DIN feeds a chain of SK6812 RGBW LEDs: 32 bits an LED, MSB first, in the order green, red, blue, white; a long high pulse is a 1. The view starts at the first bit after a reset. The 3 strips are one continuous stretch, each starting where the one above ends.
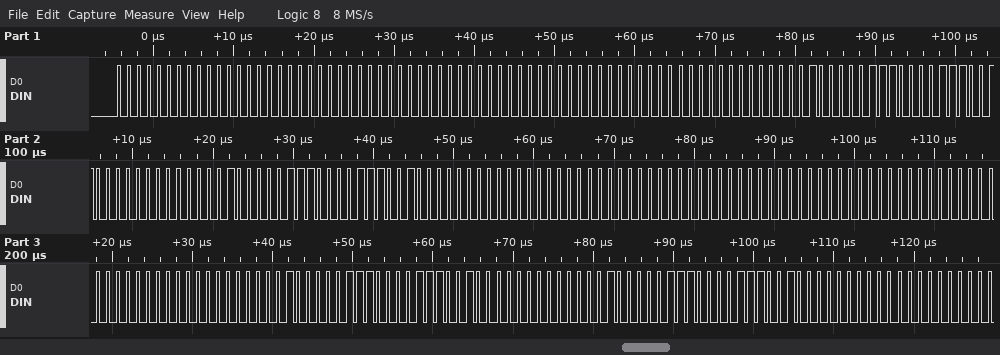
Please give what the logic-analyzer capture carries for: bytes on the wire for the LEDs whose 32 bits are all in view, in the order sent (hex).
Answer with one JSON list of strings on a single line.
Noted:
["00 00 00 00 00 00 00 00 04 1C 39 00 04 1C 39 00 00 00 00 00 00 00 00 00 04 1C 39 00 04 1C 39 00"]
